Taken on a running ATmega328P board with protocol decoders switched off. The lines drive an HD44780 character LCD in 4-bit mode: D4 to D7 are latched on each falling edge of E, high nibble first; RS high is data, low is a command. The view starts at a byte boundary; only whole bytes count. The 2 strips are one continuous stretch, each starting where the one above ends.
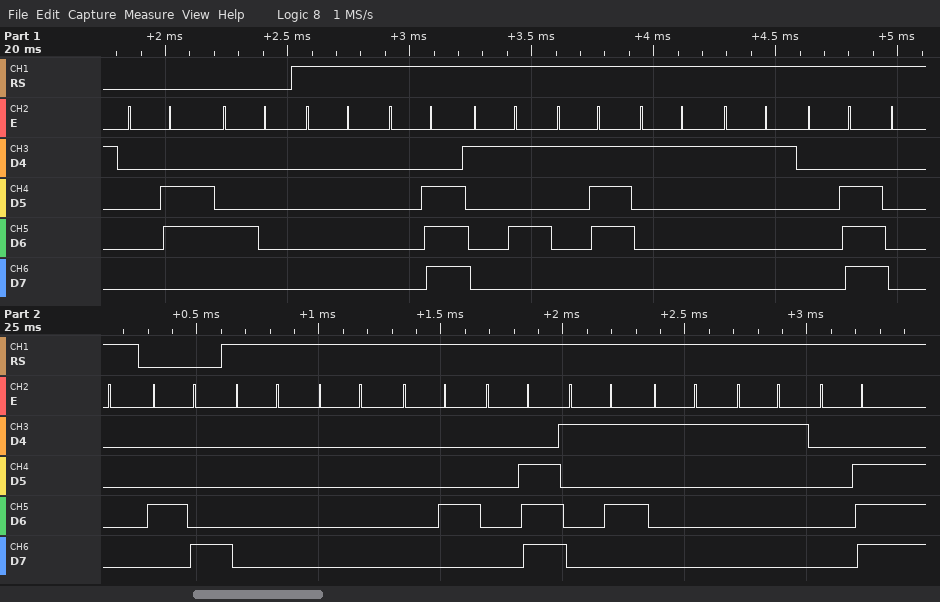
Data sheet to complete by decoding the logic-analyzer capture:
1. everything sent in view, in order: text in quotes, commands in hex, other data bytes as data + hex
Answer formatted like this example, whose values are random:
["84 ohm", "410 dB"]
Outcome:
["0x06 0x40 data 00 0E 15 17 11 11 0E 00 0x48 data 00 00 04 0E 15 11 11 0E"]
